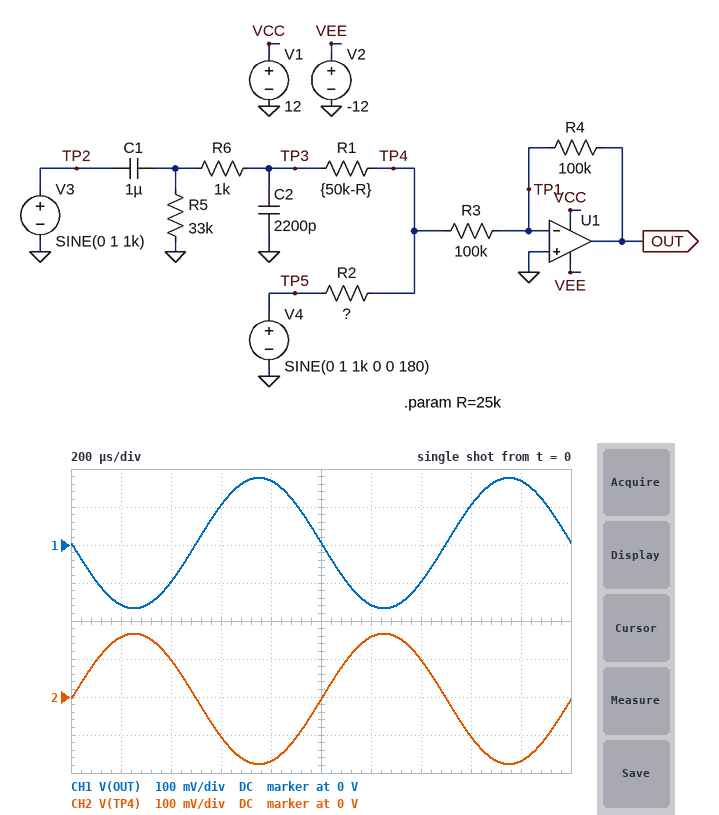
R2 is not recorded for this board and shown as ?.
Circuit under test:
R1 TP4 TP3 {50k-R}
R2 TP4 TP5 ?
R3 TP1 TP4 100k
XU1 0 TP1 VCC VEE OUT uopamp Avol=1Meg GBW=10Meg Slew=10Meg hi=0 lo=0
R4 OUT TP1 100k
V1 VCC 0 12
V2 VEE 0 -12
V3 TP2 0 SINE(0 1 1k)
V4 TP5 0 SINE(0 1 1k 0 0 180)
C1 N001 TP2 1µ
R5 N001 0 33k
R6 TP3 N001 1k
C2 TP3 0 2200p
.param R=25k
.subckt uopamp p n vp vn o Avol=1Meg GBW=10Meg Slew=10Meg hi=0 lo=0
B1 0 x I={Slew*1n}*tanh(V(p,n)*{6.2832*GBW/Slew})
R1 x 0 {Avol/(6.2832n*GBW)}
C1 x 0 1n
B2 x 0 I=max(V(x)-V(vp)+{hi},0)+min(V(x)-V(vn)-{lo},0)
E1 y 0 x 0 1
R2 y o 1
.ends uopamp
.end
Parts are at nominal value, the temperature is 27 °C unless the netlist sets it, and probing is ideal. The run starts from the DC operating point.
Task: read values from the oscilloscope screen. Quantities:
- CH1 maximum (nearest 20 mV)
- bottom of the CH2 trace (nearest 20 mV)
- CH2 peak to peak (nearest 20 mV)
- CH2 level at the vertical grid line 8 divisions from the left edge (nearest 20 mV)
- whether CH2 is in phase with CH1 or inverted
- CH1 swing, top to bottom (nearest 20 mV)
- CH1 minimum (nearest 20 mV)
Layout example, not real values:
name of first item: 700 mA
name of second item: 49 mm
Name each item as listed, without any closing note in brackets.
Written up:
CH1 maximum: 180 mV
bottom of the CH2 trace: -180 mV
CH2 peak to peak: 340 mV
CH2 level at the vertical grid line 8 divisions from the left edge: -100 mV
whether CH2 is in phase with CH1 or inverted: inverted
CH1 swing, top to bottom: 340 mV
CH1 minimum: -160 mV
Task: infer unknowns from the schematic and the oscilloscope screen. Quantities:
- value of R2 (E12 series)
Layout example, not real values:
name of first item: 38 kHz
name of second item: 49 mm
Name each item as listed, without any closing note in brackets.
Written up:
value of R2: 39 kΩ
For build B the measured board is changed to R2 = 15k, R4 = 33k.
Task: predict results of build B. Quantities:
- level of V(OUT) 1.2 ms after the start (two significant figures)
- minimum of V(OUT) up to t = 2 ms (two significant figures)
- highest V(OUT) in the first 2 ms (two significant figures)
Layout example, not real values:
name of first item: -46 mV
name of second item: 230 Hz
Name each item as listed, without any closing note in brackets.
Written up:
level of V(OUT) 1.2 ms after the start: 78 mV
minimum of V(OUT) up to t = 2 ms: -80 mV
highest V(OUT) in the first 2 ms: 82 mV
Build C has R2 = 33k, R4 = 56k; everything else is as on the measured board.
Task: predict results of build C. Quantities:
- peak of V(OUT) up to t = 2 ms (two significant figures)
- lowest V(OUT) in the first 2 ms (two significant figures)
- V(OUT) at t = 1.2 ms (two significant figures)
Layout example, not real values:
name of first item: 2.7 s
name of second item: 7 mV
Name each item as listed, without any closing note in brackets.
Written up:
peak of V(OUT) up to t = 2 ms: 60 mV
lowest V(OUT) in the first 2 ms: -55 mV
V(OUT) at t = 1.2 ms: -52 mV
